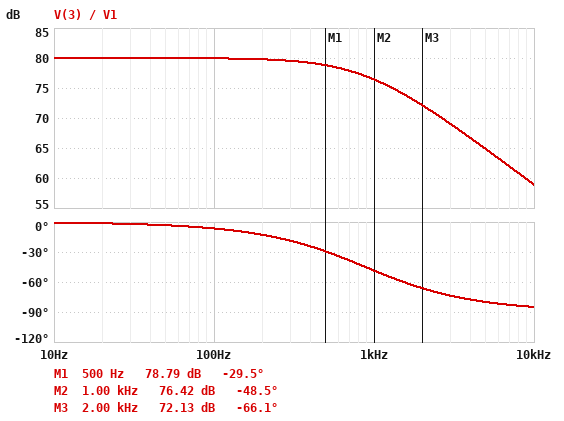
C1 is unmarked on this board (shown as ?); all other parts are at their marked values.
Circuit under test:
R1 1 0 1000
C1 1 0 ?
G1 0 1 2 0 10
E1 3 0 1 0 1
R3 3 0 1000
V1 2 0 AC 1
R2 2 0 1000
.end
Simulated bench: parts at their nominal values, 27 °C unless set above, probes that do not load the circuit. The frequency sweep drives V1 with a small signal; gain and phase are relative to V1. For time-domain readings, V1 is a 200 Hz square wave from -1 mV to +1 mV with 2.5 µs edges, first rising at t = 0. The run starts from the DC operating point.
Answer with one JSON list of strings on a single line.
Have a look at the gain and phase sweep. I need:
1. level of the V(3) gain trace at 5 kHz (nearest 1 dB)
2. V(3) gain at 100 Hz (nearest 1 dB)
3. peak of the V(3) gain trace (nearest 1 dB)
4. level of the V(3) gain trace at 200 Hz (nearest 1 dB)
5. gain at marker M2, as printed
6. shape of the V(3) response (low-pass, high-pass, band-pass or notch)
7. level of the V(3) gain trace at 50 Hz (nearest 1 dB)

["65 dB", "80 dB", "80 dB", "80 dB", "76.42 dB", "low-pass", "80 dB"]
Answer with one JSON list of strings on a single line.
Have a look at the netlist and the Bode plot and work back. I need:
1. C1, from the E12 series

["180 nF"]
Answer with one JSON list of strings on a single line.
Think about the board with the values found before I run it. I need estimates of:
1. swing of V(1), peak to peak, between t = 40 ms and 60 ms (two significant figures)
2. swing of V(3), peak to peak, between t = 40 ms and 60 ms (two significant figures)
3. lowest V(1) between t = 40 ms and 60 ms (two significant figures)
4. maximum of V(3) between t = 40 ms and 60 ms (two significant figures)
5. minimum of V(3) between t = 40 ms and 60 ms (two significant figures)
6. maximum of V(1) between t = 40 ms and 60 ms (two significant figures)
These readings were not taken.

["20 V", "20 V", "-10 V", "10 V", "-10 V", "10 V"]
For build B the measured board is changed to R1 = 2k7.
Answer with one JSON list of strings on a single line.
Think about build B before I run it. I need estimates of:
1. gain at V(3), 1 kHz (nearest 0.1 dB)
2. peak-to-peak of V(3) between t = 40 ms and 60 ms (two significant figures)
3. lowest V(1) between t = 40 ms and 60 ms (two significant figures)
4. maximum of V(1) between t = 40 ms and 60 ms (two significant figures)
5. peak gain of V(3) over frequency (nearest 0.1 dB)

["78.5 dB", "53 V", "-27 V", "27 V", "88.6 dB"]
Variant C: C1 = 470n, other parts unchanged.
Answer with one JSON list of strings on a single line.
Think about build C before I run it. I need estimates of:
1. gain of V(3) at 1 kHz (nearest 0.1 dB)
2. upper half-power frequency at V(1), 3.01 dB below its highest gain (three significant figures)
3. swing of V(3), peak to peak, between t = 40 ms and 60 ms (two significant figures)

["70.1 dB", "339 Hz", "20 V"]
